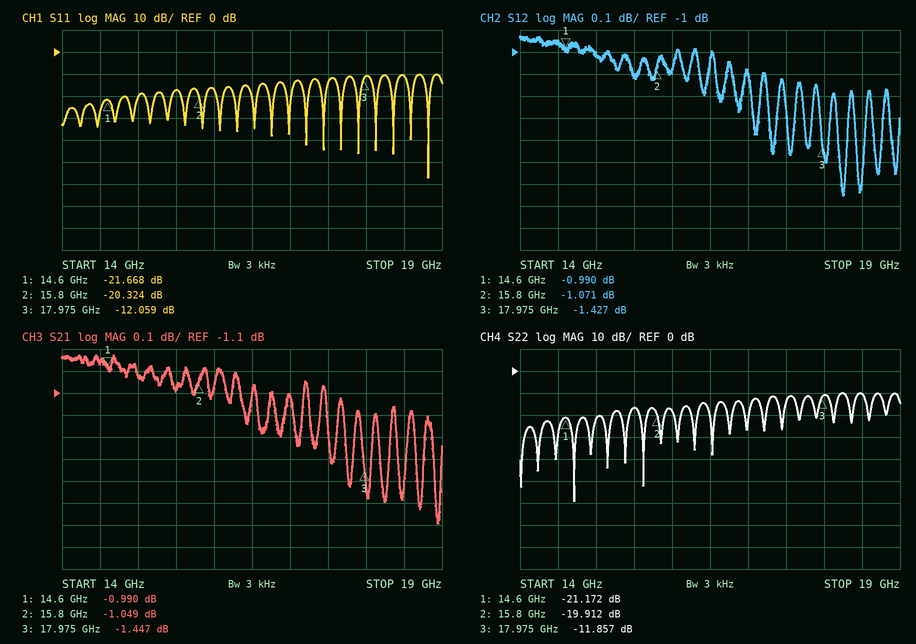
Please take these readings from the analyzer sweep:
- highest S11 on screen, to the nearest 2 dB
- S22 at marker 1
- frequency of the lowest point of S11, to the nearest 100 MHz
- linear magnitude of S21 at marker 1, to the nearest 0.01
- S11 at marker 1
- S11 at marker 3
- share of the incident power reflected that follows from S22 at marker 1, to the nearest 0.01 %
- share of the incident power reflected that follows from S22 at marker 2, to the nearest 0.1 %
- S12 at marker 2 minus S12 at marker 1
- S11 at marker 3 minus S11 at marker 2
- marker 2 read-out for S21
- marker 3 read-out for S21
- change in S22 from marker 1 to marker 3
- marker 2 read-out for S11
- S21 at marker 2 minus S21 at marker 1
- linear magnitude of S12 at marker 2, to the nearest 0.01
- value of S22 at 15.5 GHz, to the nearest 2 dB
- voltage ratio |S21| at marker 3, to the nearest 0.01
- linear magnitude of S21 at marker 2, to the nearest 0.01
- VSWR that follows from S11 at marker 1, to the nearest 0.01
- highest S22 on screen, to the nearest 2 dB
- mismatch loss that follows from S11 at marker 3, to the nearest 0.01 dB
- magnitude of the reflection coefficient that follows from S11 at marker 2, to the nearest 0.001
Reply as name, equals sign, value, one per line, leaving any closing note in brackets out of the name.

highest S11 on screen, to the nearest 2 dB = -10 dB
S22 at marker 1 = -21.172 dB
frequency of the lowest point of S11, to the nearest 100 MHz = 18.8 GHz
linear magnitude of S21 at marker 1, to the nearest 0.01 = 0.89
S11 at marker 1 = -21.668 dB
S11 at marker 3 = -12.059 dB
share of the incident power reflected that follows from S22 at marker 1, to the nearest 0.01 % = 0.76 %
share of the incident power reflected that follows from S22 at marker 2, to the nearest 0.1 % = 1.0 %
S12 at marker 2 minus S12 at marker 1 = -0.081 dB
S11 at marker 3 minus S11 at marker 2 = 8.265 dB
marker 2 read-out for S21 = -1.049 dB
marker 3 read-out for S21 = -1.447 dB
change in S22 from marker 1 to marker 3 = 9.315 dB
marker 2 read-out for S11 = -20.324 dB
S21 at marker 2 minus S21 at marker 1 = -0.059 dB
linear magnitude of S12 at marker 2, to the nearest 0.01 = 0.88
value of S22 at 15.5 GHz, to the nearest 2 dB = -16 dB
voltage ratio |S21| at marker 3, to the nearest 0.01 = 0.85
linear magnitude of S21 at marker 2, to the nearest 0.01 = 0.89
VSWR that follows from S11 at marker 1, to the nearest 0.01 = 1.18
highest S22 on screen, to the nearest 2 dB = -10 dB
mismatch loss that follows from S11 at marker 3, to the nearest 0.01 dB = 0.28 dB
magnitude of the reflection coefficient that follows from S11 at marker 2, to the nearest 0.001 = 0.096
